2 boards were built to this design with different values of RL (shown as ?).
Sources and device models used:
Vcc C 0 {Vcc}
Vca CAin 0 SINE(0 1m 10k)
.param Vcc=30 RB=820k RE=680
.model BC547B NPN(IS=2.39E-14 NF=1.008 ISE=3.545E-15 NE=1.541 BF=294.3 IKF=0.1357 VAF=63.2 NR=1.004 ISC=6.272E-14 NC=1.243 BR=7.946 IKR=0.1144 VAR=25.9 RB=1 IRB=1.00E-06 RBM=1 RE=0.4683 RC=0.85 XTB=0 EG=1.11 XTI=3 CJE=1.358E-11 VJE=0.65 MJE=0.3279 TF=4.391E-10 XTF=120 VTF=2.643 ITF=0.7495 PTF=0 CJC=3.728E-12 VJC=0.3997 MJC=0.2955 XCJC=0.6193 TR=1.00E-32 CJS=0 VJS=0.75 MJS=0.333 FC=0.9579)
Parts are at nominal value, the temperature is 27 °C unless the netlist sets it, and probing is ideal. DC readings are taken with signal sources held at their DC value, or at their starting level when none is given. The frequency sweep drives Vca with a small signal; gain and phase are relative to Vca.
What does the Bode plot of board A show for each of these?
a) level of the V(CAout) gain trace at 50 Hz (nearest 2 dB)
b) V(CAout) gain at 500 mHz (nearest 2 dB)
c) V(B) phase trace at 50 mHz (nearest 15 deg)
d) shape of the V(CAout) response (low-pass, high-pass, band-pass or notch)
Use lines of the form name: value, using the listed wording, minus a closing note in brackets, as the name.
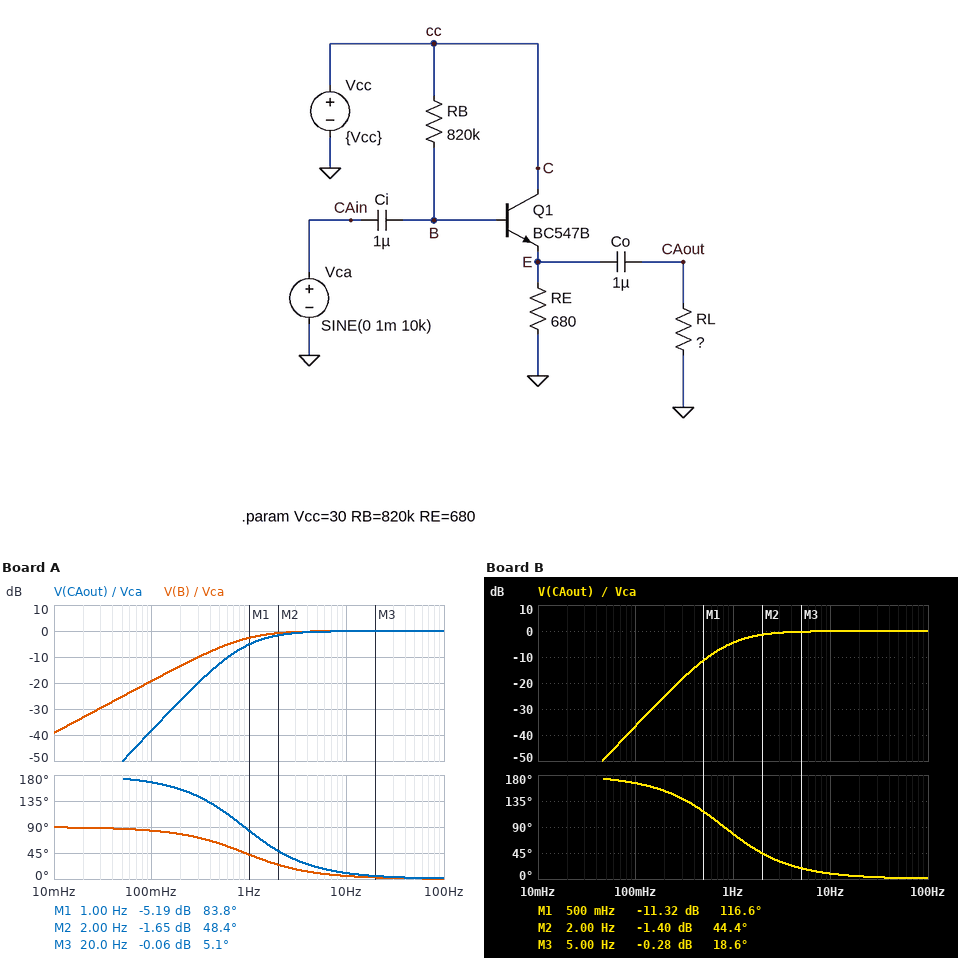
level of the V(CAout) gain trace at 50 Hz: 0 dB
V(CAout) gain at 500 mHz: -12 dB
V(B) phase trace at 50 mHz: 90 deg
shape of the V(CAout) response: high-pass
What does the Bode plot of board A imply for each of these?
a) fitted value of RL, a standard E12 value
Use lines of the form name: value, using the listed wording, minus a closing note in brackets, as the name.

fitted value of RL, a standard E12 value: 180 kΩ
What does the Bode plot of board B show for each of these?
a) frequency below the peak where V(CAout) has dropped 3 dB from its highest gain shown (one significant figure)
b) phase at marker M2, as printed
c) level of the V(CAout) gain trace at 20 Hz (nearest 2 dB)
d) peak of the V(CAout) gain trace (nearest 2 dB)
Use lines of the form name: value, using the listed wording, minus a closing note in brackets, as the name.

frequency below the peak where V(CAout) has dropped 3 dB from its highest gain shown: 1 Hz
phase at marker M2, as printed: 44.4 deg
level of the V(CAout) gain trace at 20 Hz: 0 dB
peak of the V(CAout) gain trace: 0 dB
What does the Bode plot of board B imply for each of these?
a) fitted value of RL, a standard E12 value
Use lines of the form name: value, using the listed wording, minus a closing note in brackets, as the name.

fitted value of RL, a standard E12 value: 220 kΩ
